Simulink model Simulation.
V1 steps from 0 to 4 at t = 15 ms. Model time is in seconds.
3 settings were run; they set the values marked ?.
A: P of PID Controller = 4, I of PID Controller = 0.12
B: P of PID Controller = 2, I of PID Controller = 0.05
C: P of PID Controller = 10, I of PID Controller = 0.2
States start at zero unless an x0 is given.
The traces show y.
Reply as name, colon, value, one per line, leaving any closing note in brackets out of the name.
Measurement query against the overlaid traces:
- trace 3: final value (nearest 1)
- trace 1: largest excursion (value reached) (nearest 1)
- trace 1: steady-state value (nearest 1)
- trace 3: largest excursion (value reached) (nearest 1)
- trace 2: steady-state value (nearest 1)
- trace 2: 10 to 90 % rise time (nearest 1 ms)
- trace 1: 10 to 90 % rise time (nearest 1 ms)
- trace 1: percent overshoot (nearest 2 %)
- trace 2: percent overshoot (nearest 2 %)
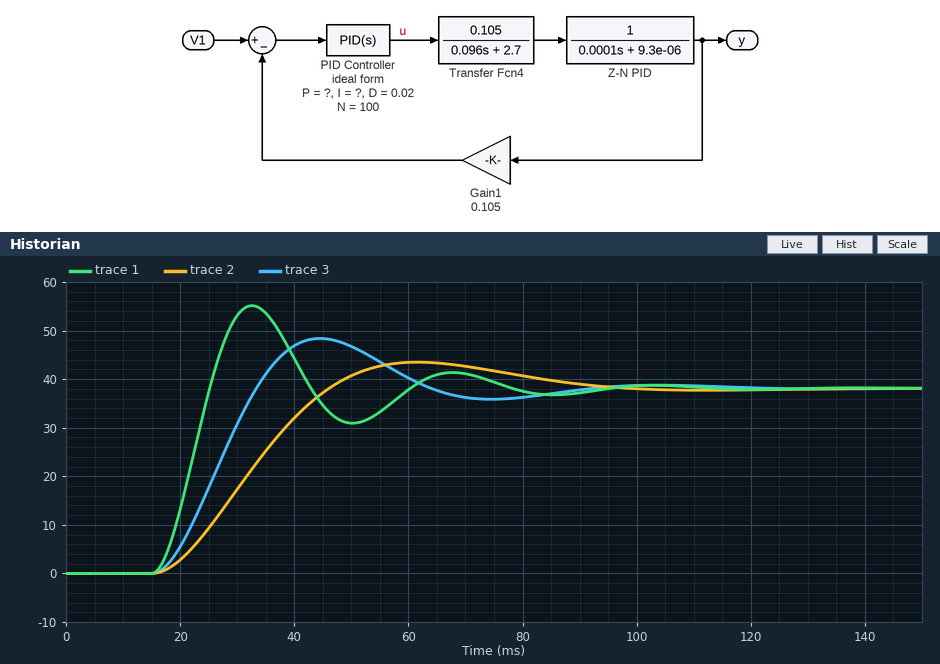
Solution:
trace 3: final value: 38
trace 1: largest excursion (value reached): 55
trace 1: steady-state value: 38
trace 3: largest excursion (value reached): 48
trace 2: steady-state value: 38
trace 2: 10 to 90 % rise time: 21 ms
trace 1: 10 to 90 % rise time: 7 ms
trace 1: percent overshoot: 44 %
trace 2: percent overshoot: 14 %
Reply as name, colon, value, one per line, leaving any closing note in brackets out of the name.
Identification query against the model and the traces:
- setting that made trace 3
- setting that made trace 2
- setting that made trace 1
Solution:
setting that made trace 3: A
setting that made trace 2: B
setting that made trace 1: C
